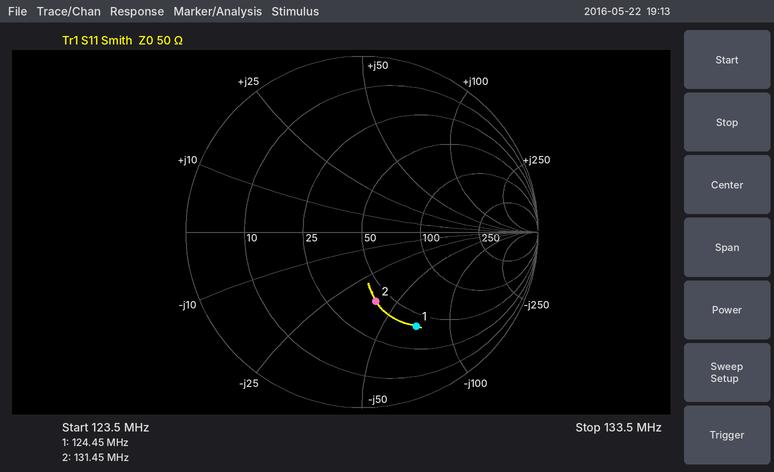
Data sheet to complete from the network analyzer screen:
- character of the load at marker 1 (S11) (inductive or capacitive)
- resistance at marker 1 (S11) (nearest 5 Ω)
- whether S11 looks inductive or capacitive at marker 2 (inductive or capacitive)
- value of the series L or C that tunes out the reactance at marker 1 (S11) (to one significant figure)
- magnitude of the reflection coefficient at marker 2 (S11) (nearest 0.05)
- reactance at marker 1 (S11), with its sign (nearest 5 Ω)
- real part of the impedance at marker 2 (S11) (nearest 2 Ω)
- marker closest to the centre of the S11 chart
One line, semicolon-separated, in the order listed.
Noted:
capacitive; 40 Ω; capacitive; 90 nH; 0.40; -70 Ω; 42 Ω; marker 2
